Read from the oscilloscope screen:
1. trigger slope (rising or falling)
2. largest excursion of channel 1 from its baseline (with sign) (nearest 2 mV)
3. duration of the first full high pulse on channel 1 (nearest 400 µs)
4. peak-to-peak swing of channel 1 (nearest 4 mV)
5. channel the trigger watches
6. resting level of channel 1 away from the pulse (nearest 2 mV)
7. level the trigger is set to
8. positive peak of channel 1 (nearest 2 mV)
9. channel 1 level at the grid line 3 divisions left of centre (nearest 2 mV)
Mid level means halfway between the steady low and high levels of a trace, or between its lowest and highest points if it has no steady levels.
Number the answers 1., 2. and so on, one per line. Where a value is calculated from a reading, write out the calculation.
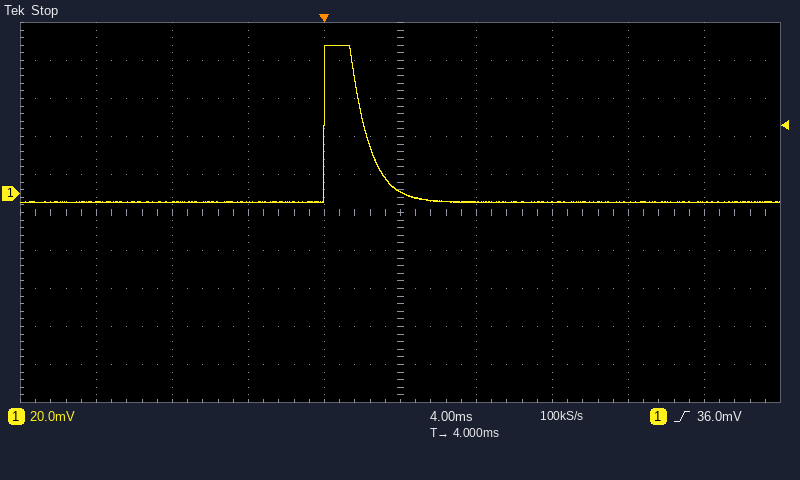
1. rising
2. 78 mV − (-4 mV) = +82 mV
3. 2.0 ms
4. 84 mV
5. channel 1
6. -4 mV
7. 36.0 mV
8. 78 mV
9. -4 mV
